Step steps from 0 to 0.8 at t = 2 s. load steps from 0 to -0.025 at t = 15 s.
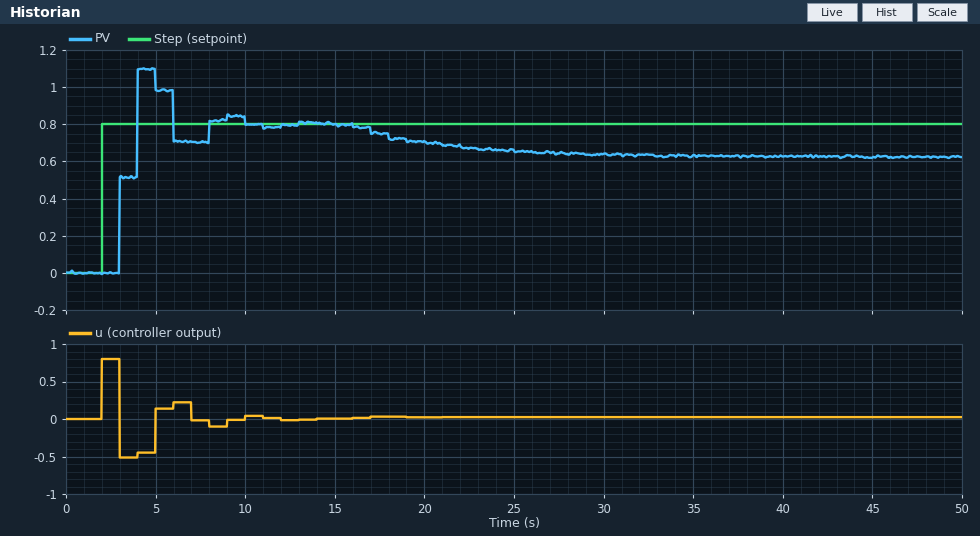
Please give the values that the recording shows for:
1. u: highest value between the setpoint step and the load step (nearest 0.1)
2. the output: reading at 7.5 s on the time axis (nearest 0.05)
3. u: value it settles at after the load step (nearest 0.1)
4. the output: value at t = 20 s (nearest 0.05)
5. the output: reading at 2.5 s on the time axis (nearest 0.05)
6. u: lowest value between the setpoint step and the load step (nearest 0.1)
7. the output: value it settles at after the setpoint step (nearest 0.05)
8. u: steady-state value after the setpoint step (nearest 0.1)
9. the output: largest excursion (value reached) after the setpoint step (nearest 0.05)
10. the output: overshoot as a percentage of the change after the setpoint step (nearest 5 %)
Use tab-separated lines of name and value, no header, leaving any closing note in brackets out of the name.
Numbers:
u: highest value between the setpoint step and the load step	0.8
the output: reading at 7.5 s on the time axis	0.70
u: value it settles at after the load step	0.0
the output: value at t = 20 s	0.70
the output: reading at 2.5 s on the time axis	0.00
u: lowest value between the setpoint step and the load step	-0.5
the output: value it settles at after the setpoint step	0.80
u: steady-state value after the setpoint step	0.0
the output: largest excursion (value reached) after the setpoint step	1.10
the output: overshoot as a percentage of the change after the setpoint step	35 %
